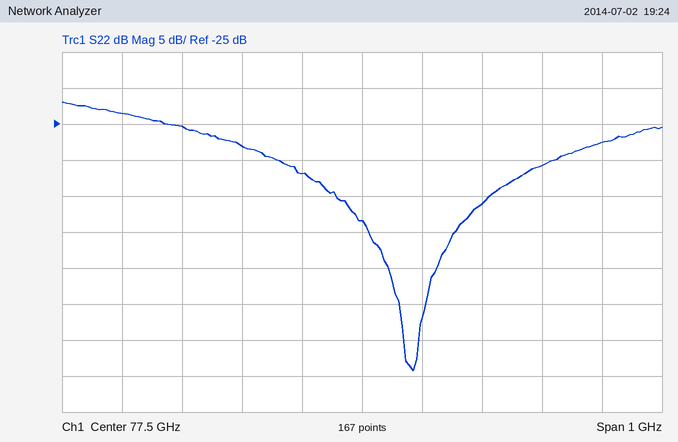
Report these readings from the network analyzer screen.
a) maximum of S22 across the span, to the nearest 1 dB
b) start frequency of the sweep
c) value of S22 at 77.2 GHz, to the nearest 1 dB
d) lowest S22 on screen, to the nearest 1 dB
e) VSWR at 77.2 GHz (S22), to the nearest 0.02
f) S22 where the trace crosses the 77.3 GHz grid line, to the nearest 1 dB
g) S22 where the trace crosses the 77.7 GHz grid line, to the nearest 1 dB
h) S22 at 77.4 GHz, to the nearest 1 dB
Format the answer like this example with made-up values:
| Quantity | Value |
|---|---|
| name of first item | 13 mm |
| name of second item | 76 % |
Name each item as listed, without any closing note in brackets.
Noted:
| Quantity | Value |
|---|---|
| maximum of S22 across the span, to the nearest 1 dB | -22 dB |
| start frequency of the sweep | 77 GHz |
| value of S22 at 77.2 GHz, to the nearest 1 dB | -25 dB |
| lowest S22 on screen, to the nearest 1 dB | -59 dB |
| VSWR at 77.2 GHz (S22), to the nearest 0.02 | 1.12 |
| S22 where the trace crosses the 77.3 GHz grid line, to the nearest 1 dB | -28 dB |
| S22 where the trace crosses the 77.7 GHz grid line, to the nearest 1 dB | -36 dB |
| S22 at 77.4 GHz, to the nearest 1 dB | -32 dB |
